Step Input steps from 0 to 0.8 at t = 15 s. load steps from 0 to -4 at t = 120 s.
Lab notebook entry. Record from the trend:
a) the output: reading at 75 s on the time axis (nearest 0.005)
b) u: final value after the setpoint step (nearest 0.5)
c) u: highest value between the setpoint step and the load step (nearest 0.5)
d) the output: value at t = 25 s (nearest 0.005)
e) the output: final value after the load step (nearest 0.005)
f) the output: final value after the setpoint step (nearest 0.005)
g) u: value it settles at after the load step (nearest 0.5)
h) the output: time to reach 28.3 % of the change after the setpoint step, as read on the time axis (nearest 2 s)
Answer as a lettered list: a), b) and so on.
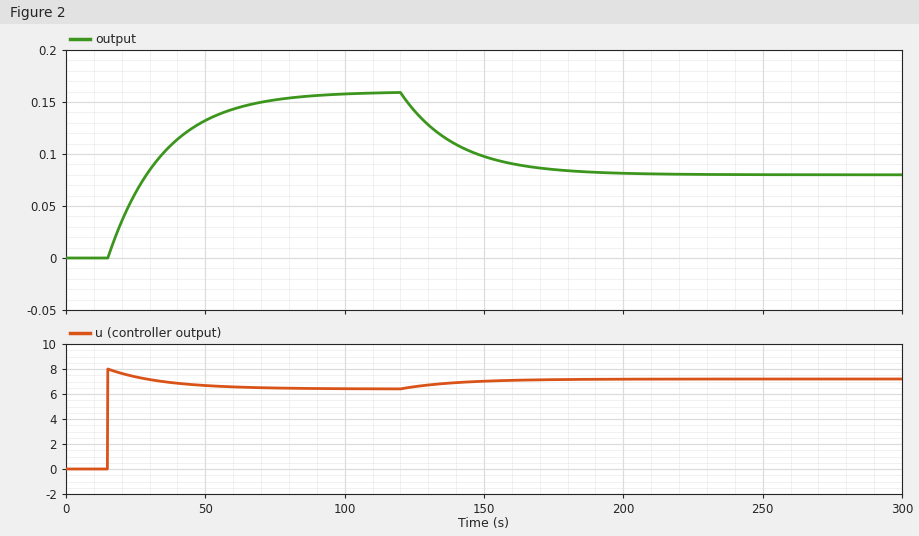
a) 0.150
b) 6.5
c) 8.0
d) 0.065
e) 0.080
f) 0.160
g) 7.0
h) 22 s
